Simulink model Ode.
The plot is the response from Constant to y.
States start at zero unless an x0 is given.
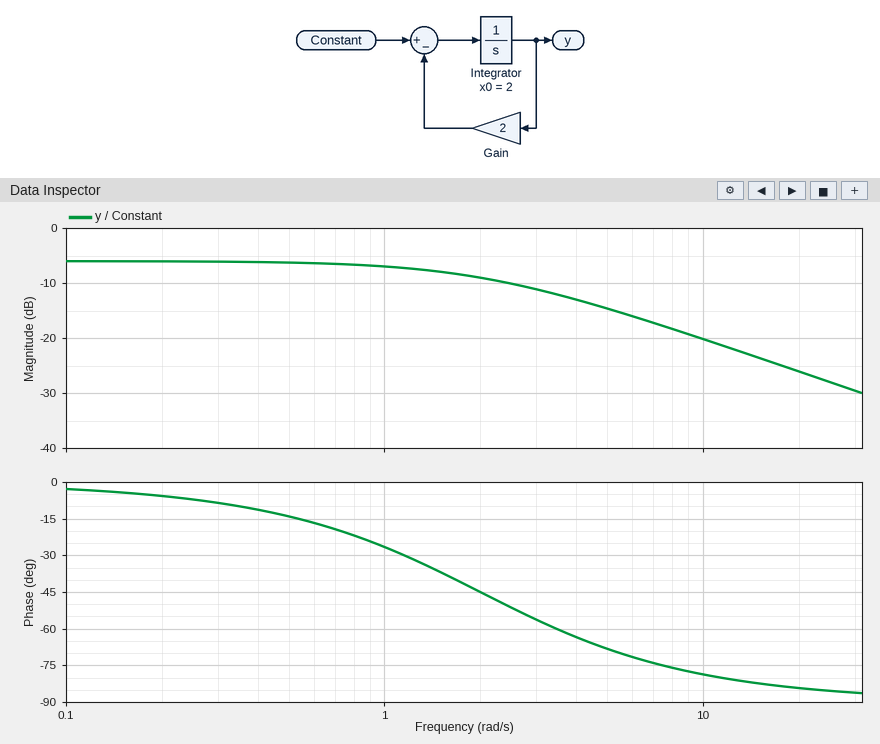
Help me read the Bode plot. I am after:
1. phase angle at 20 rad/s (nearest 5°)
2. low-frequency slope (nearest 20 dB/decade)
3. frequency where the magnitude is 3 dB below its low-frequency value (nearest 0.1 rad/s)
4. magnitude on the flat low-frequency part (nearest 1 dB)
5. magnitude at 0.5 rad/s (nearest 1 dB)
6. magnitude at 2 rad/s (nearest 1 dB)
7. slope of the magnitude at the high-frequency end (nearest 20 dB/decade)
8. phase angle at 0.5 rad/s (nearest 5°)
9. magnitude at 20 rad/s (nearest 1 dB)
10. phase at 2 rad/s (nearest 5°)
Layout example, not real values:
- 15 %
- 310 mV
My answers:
- -85°
- 0 dB/decade
- 2.0 rad/s
- -6 dB
- -6 dB
- -9 dB
- -20 dB/decade
- -15°
- -26 dB
- -45°
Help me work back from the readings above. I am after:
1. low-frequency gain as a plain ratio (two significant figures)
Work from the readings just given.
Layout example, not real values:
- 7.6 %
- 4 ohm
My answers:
- 0.50
